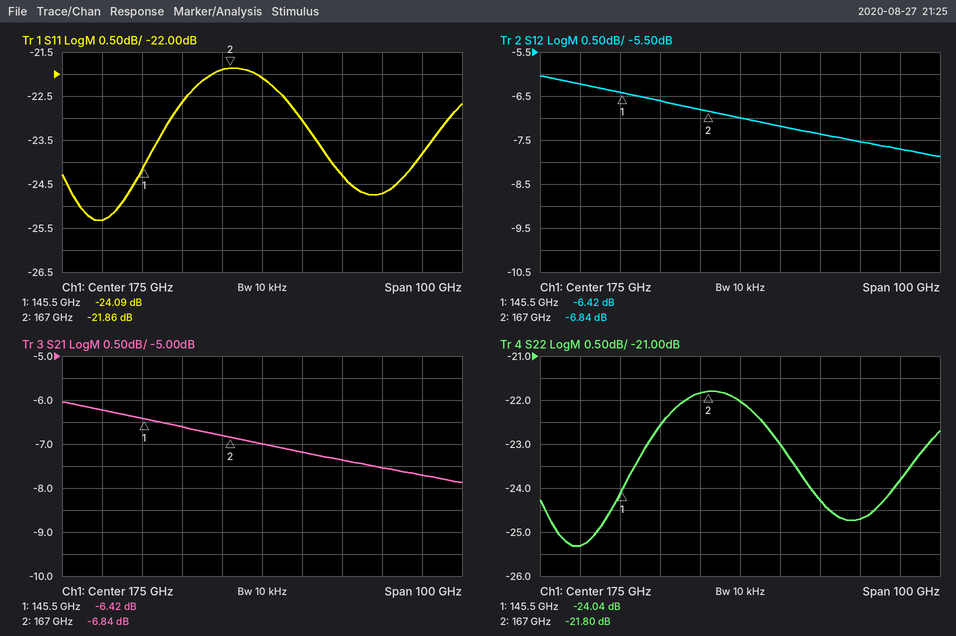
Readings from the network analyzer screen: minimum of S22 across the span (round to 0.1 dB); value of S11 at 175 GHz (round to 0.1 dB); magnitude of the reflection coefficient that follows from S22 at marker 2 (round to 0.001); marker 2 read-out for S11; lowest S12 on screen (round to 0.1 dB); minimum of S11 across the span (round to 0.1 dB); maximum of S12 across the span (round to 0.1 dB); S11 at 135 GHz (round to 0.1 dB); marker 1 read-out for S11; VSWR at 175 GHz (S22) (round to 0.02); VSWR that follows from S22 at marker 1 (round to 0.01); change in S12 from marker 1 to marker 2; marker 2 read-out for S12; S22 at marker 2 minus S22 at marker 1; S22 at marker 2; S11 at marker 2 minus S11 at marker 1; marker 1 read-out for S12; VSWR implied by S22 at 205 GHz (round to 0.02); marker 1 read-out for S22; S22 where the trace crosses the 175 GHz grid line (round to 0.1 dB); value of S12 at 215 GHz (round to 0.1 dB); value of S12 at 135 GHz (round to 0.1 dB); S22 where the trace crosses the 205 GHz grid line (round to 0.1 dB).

-25.3 dB
-22.1 dB
0.081
-21.86 dB
-7.9 dB
-25.3 dB
-6.0 dB
-25.3 dB
-24.09 dB
1.18
1.13
-0.42 dB
-6.84 dB
2.24 dB
-21.80 dB
2.23 dB
-6.42 dB
1.12
-24.04 dB
-22.0 dB
-7.7 dB
-6.2 dB
-24.7 dB
